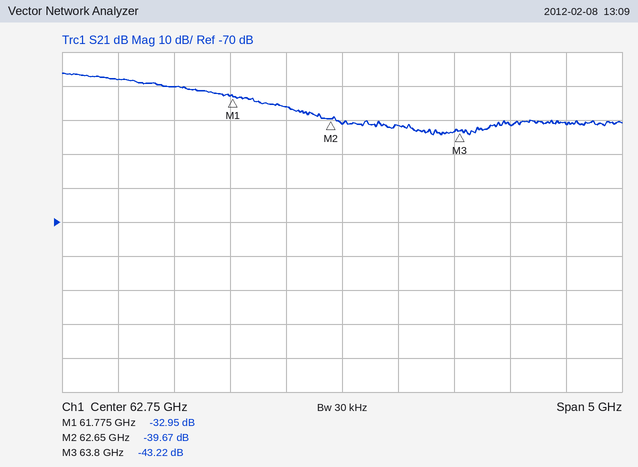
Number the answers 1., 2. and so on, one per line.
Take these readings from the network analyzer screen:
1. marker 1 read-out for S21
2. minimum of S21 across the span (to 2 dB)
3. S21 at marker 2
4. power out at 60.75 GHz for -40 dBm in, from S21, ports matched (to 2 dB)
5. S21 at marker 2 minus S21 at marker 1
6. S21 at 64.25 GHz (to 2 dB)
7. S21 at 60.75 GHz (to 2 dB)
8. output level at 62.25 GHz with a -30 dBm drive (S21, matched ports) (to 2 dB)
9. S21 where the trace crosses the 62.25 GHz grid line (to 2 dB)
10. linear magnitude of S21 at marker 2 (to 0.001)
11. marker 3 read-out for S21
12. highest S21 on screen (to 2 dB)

1. -32.95 dB
2. -44 dB
3. -39.67 dB
4. -68 dBm
5. -6.72 dB
6. -42 dB
7. -28 dB
8. -66 dBm
9. -36 dB
10. 0.010
11. -43.22 dB
12. -26 dB
